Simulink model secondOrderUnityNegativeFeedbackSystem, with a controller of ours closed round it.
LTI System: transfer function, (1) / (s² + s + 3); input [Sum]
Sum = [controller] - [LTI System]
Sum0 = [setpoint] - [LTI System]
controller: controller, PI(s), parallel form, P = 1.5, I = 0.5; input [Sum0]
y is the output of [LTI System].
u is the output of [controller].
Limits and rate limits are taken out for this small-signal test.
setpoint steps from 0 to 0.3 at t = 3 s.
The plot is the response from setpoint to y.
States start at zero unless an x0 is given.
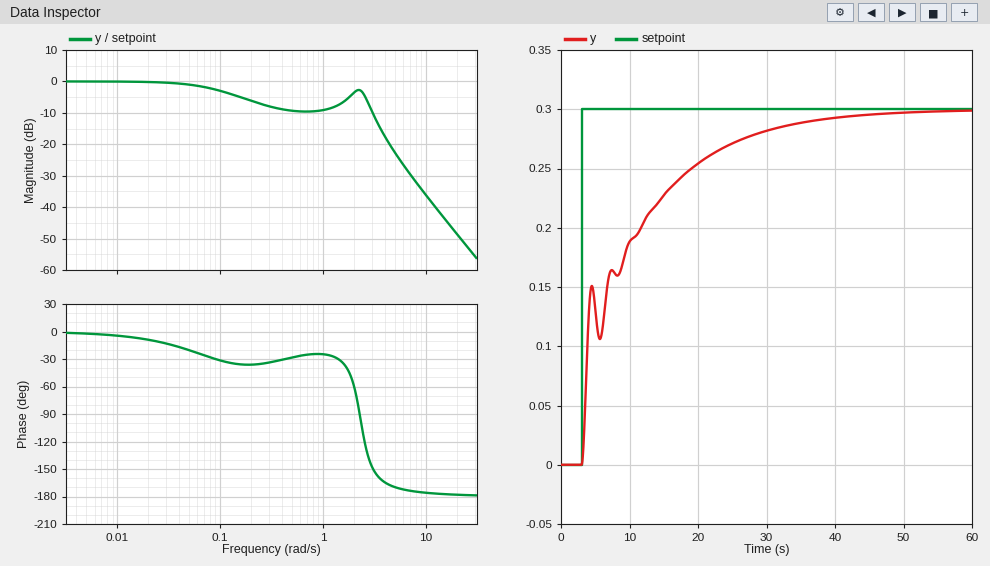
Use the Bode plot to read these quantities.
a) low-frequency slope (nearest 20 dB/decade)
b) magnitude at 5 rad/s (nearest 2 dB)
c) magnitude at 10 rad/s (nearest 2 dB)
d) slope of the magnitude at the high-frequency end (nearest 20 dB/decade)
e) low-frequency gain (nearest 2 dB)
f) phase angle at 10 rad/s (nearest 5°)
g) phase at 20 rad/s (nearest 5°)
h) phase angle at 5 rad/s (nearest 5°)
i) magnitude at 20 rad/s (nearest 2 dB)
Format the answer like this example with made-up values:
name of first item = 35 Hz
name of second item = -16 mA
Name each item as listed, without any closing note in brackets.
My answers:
low-frequency slope = 0 dB/decade
magnitude at 5 rad/s = -22 dB
magnitude at 10 rad/s = -36 dB
slope of the magnitude at the high-frequency end = -40 dB/decade
low-frequency gain = 0 dB
phase angle at 10 rad/s = -175°
phase at 20 rad/s = -180°
phase angle at 5 rad/s = -170°
magnitude at 20 rad/s = -48 dB
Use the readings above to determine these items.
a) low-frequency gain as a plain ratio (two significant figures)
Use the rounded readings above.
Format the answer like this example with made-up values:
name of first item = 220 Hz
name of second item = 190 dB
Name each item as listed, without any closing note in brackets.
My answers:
low-frequency gain as a plain ratio = 1.0
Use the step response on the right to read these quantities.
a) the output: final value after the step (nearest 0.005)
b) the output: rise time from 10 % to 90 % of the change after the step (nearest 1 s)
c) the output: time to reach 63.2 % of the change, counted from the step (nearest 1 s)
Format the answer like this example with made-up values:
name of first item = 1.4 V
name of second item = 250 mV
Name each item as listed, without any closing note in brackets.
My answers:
the output: final value after the step = 0.300
the output: rise time from 10 % to 90 % of the change after the step = 21 s
the output: time to reach 63.2 % of the change, counted from the step = 7 s
